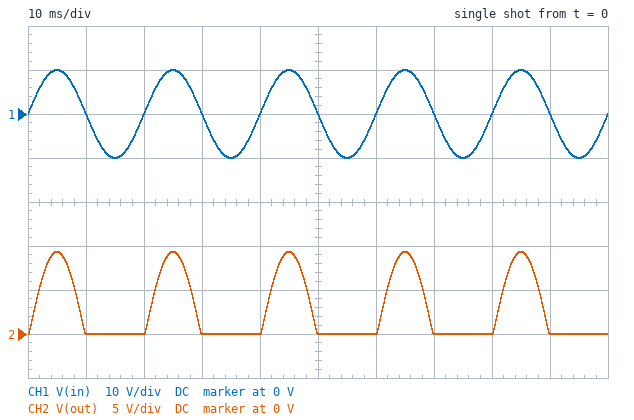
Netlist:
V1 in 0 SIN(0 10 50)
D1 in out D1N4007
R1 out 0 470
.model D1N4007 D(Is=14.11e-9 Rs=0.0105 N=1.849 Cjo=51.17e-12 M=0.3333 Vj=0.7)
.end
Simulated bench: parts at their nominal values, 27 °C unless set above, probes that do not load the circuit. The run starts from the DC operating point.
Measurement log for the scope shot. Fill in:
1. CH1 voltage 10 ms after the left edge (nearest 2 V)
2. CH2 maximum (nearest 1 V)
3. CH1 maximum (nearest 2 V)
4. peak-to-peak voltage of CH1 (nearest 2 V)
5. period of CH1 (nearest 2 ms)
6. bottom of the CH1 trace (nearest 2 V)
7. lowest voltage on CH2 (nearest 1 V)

0 V
9 V
10 V
20 V
20 ms
-10 V
0 V
